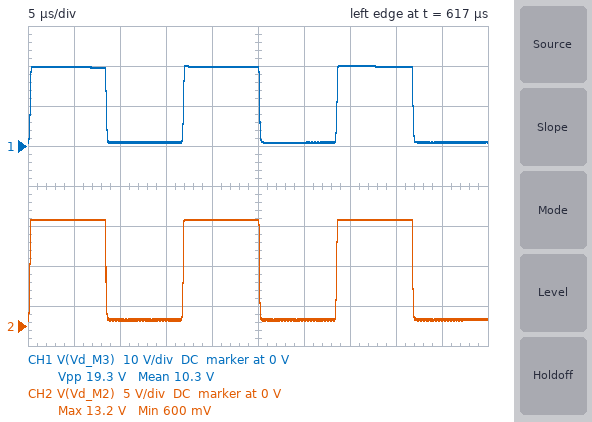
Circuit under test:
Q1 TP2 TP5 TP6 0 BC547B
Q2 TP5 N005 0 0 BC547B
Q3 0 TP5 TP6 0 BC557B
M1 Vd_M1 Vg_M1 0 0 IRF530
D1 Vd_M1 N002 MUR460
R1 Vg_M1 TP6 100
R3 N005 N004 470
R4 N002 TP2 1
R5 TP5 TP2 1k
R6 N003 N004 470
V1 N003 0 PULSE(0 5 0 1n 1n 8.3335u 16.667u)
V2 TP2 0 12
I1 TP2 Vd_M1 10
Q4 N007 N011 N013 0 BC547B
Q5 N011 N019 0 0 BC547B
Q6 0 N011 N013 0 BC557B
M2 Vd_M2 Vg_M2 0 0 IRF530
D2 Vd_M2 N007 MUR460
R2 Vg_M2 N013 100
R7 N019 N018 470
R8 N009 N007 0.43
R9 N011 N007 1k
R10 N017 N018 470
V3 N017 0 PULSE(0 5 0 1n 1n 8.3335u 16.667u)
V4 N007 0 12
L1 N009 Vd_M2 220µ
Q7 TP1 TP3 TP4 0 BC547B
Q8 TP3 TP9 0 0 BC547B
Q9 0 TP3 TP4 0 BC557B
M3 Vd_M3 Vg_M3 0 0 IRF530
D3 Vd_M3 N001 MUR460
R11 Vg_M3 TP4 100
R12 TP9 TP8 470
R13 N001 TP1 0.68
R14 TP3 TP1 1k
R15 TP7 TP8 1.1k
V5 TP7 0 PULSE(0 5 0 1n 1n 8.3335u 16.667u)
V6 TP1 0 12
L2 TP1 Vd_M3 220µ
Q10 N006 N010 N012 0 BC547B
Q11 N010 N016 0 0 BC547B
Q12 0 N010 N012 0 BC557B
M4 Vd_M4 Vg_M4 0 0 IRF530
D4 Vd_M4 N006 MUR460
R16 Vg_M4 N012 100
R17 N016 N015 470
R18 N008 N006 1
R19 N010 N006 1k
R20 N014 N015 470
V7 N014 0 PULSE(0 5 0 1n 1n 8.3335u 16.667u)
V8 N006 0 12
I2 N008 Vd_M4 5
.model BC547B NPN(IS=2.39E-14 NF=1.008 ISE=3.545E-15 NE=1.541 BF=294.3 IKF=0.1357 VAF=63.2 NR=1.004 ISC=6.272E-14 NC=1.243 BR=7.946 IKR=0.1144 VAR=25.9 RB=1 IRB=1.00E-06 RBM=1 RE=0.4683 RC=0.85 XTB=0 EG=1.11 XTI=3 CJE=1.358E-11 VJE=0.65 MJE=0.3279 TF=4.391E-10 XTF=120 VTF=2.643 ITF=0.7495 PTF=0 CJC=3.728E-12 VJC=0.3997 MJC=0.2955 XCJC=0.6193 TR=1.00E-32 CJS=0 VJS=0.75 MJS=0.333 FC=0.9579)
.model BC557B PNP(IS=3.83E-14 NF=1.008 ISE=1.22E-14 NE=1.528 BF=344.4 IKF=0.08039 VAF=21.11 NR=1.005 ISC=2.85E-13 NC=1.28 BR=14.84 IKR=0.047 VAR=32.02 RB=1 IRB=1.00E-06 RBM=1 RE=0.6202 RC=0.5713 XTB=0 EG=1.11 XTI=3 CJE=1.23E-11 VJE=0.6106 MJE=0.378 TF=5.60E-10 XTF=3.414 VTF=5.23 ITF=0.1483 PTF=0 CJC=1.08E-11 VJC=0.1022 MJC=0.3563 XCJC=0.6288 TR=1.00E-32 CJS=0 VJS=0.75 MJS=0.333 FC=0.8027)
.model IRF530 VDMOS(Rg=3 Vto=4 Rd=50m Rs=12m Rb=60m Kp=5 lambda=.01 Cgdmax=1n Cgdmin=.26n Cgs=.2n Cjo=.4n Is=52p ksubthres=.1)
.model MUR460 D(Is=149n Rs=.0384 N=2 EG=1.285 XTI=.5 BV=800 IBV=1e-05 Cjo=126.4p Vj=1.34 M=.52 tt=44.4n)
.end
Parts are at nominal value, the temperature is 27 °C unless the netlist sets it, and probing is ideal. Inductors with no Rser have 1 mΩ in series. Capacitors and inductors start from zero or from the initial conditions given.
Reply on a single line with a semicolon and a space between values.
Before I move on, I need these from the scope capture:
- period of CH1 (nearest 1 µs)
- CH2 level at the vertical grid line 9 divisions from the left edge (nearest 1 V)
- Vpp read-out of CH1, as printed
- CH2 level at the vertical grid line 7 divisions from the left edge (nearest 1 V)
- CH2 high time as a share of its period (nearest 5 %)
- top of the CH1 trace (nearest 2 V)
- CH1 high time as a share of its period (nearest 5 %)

17 µs; 1 V; 19.3 V; 13 V; 50 %; 20 V; 50 %
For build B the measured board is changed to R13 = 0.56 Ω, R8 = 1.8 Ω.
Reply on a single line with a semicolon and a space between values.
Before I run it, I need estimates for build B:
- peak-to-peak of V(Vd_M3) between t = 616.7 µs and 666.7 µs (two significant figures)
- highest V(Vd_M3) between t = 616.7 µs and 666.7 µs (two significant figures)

18 V; 19 V
